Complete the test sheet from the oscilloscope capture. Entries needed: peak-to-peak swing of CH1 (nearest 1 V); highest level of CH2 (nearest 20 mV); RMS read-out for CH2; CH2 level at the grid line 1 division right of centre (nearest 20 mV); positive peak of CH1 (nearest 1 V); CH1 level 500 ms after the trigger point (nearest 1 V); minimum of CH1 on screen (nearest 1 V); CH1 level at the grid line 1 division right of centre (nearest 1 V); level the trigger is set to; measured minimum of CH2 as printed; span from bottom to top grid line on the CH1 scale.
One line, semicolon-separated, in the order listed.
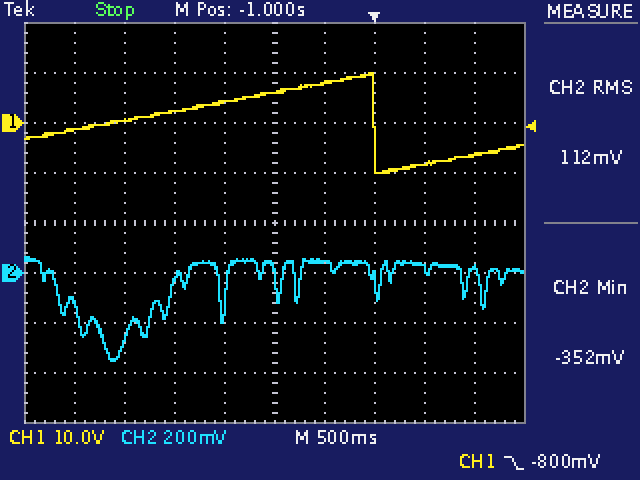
20 V; 60 mV; 112 mV; 40 mV; 10 V; -8 V; -10 V; 8 V; -800 mV; -352 mV; 80 V
